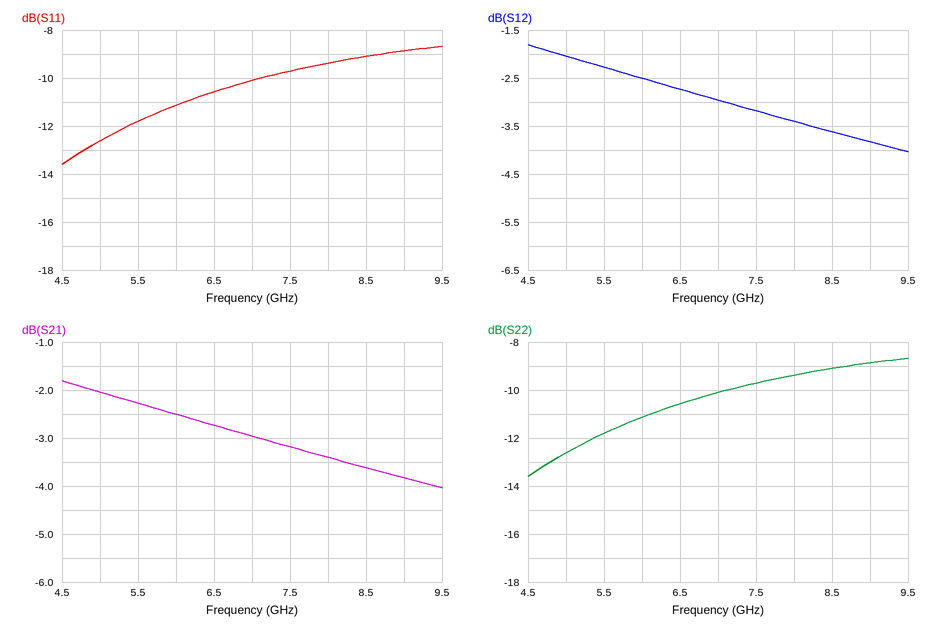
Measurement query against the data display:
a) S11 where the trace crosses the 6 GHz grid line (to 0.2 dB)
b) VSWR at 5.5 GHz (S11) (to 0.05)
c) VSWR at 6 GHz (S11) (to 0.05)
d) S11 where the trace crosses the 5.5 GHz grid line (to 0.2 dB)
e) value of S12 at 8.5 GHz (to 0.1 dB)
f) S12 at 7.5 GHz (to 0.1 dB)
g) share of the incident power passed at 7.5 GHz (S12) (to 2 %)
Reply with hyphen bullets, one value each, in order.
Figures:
- -11.2 dB
- 1.70
- 1.75
- -11.8 dB
- -3.6 dB
- -3.2 dB
- 48 %
